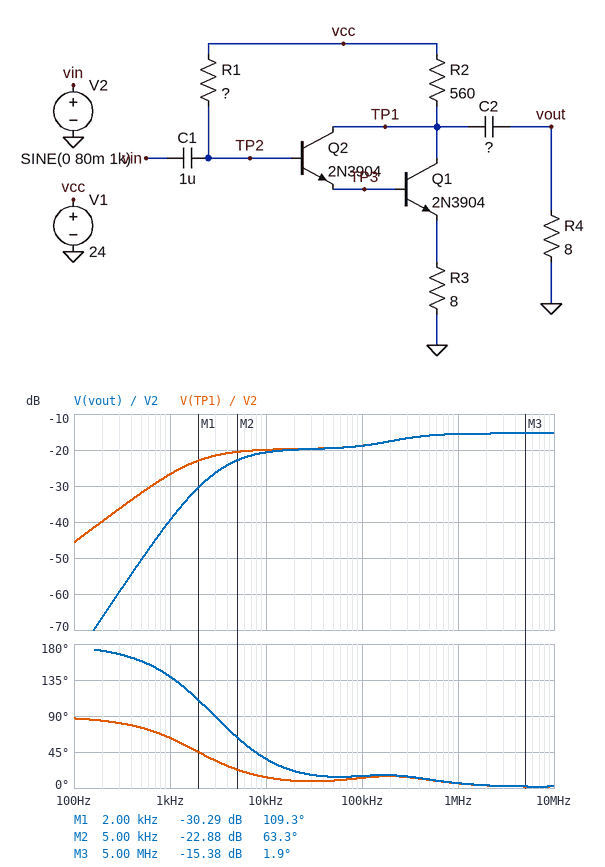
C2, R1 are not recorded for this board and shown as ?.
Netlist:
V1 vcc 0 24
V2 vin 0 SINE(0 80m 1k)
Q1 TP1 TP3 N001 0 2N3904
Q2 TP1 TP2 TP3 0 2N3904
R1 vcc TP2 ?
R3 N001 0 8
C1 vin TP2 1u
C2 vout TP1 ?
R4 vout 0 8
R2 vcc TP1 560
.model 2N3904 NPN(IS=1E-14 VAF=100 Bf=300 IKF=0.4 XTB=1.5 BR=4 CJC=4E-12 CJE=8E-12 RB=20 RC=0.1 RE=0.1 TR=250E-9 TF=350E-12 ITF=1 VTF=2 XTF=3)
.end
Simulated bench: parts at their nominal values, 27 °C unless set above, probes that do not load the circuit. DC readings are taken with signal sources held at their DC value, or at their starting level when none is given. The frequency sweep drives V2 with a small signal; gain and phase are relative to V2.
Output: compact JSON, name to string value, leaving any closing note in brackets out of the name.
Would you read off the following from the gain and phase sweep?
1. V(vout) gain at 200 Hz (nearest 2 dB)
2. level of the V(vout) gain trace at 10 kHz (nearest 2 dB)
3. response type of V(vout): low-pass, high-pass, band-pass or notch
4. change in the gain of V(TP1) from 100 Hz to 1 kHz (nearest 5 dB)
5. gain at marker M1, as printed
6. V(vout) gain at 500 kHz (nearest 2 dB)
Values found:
{"V(vout) gain at 200 Hz": "-66 dB", "level of the V(vout) gain trace at 10 kHz": "-20 dB", "response type of V(vout): low-pass, high-pass, band-pass or notch": "high-pass", "change in the gain of V(TP1) from 100 Hz to 1 kHz": "20 dB", "gain at marker M1, as printed": "-30.29 dB", "V(vout) gain at 500 kHz": "-16 dB"}
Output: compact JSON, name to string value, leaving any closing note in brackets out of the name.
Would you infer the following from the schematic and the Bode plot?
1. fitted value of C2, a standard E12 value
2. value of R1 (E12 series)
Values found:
{"fitted value of C2, a standard E12 value": "4.7 µF", "value of R1": "12 kΩ"}
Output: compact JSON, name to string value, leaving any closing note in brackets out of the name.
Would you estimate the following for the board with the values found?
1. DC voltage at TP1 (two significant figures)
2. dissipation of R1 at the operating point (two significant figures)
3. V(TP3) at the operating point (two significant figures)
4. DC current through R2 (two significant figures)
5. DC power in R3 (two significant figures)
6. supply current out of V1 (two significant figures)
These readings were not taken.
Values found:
{"DC voltage at TP1": "1.1 V", "dissipation of R1 at the operating point": "41 mW", "V(TP3) at the operating point": "1.1 V", "DC current through R2": "41 mA", "DC power in R3": "15 mW", "supply current out of V1": "43 mA"}
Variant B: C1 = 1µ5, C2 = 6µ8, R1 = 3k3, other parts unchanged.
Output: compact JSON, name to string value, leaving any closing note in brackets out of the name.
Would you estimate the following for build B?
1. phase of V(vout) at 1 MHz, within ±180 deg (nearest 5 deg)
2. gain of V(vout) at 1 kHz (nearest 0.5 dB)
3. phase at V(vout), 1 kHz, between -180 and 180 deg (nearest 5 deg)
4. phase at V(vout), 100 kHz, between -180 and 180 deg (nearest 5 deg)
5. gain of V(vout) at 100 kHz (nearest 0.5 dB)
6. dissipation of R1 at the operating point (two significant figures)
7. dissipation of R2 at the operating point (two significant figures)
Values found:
{"phase of V(vout) at 1 MHz, within ±180 deg": "0 deg", "gain of V(vout) at 1 kHz": "-33.5 dB", "phase at V(vout), 1 kHz, between -180 and 180 deg": "130 deg", "phase at V(vout), 100 kHz, between -180 and 180 deg": "5 deg", "gain of V(vout) at 100 kHz": "-16.5 dB", "dissipation of R1 at the operating point": "150 mW", "dissipation of R2 at the operating point": "930 mW"}
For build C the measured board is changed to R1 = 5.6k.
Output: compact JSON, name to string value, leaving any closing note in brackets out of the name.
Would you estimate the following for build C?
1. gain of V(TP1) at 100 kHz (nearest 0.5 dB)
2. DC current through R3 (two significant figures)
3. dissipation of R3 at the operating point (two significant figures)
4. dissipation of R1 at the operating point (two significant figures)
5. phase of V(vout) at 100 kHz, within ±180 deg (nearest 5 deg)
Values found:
{"gain of V(TP1) at 100 kHz": "-17.0 dB", "DC current through R3": "45 mA", "dissipation of R3 at the operating point": "16 mW", "dissipation of R1 at the operating point": "87 mW", "phase of V(vout) at 100 kHz, within ±180 deg": "10 deg"}
